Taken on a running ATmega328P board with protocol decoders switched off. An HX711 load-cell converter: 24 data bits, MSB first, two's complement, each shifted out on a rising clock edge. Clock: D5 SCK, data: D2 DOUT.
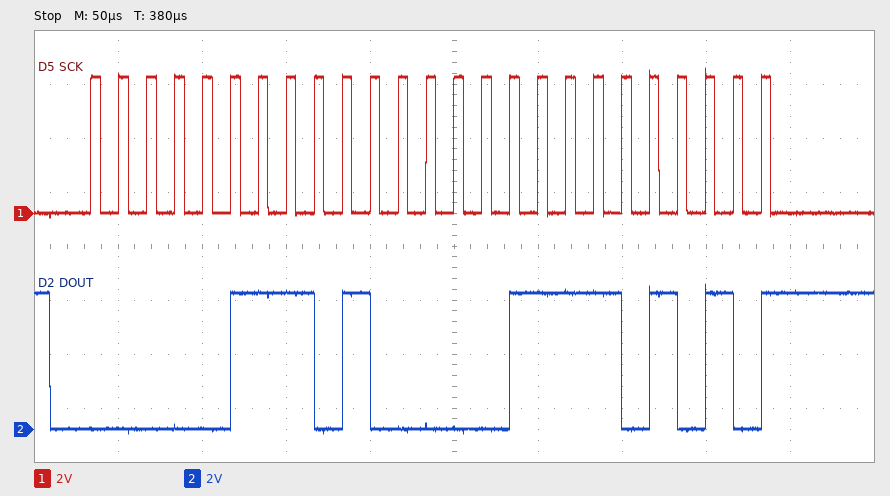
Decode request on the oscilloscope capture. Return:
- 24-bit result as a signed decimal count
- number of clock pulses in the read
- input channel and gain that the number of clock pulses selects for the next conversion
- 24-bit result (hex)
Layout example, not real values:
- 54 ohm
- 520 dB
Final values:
- 475626
- 25
- channel A, gain 128
- 0x0741EA
